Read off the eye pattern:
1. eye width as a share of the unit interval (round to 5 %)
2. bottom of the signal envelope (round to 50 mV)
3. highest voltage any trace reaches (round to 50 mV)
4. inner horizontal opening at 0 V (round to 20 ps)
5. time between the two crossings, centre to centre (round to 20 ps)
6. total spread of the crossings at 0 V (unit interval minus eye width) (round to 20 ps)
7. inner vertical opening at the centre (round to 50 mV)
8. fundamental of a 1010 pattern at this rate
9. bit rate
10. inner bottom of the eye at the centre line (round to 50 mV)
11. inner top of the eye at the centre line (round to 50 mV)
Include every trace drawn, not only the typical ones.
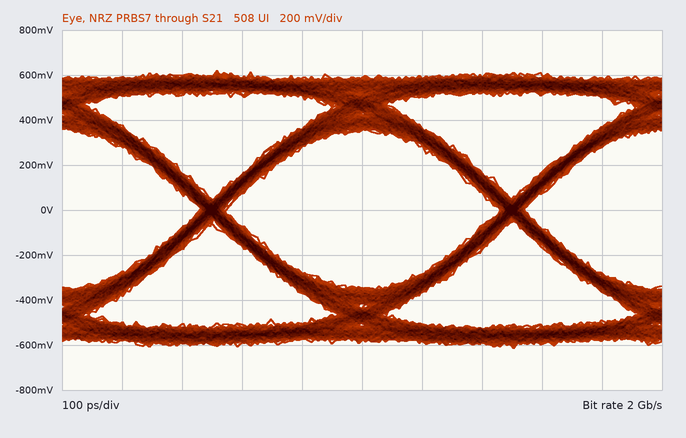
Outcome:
90 %
-600 mV
600 mV
460 ps
500 ps
40 ps
700 mV
1 GHz
2 Gb/s
-350 mV
350 mV
